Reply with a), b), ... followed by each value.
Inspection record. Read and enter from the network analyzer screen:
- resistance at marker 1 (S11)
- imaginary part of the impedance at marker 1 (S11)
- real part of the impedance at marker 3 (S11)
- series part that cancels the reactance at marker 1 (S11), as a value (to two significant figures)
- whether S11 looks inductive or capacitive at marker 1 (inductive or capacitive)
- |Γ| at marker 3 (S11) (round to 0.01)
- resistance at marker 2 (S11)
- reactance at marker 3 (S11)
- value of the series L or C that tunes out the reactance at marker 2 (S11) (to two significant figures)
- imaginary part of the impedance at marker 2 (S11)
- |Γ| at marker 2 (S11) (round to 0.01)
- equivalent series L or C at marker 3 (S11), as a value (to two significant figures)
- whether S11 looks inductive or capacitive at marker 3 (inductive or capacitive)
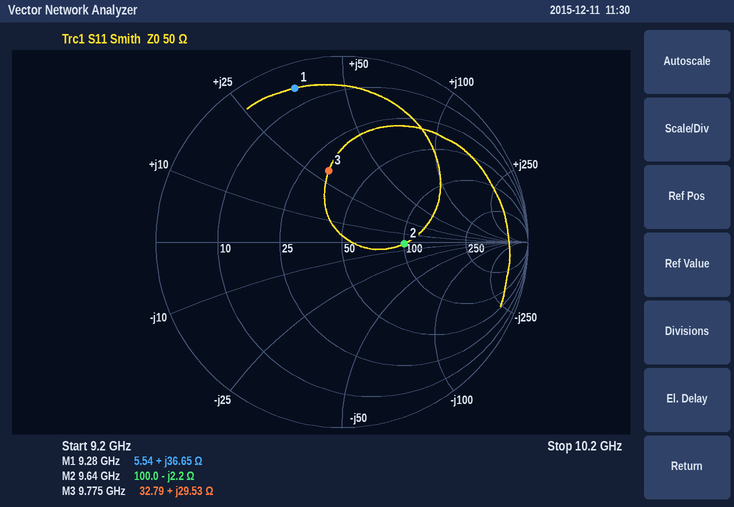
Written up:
a) 5.54 Ω
b) +36.65 Ω
c) 32.79 Ω
d) 470 fF
e) inductive
f) 0.39
g) 100.0 Ω
h) +29.53 Ω
i) 36 pH
j) -2.2 Ω
k) 0.33
l) 480 pH
m) inductive
